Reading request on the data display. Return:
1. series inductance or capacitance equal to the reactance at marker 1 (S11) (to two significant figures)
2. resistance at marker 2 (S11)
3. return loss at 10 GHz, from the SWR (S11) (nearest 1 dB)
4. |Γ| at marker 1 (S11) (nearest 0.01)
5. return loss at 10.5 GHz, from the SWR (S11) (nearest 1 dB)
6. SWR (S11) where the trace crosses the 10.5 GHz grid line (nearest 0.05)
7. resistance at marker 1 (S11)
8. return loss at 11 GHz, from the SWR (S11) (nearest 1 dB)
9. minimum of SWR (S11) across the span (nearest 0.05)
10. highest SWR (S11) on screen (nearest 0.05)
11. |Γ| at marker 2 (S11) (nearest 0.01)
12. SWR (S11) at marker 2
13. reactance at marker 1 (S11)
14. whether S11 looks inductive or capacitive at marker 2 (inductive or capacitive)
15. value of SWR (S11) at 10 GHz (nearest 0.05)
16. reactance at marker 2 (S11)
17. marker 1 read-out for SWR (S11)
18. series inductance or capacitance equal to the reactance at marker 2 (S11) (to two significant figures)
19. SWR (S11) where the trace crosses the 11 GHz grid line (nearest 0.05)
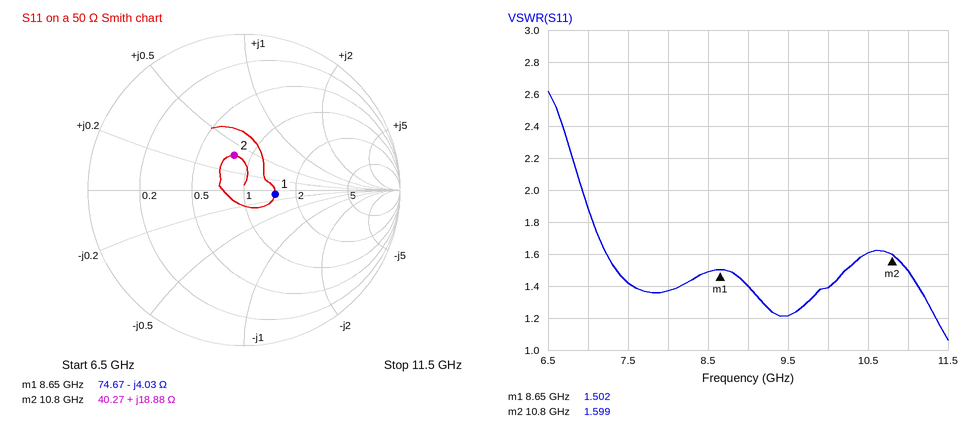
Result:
4.6 pF
40.27 Ω
16 dB
0.20
13 dB
1.60
74.67 Ω
14 dB
1.05
2.60
0.23
1.599
-4.03 Ω
inductive
1.40
+18.88 Ω
1.502
280 pH
1.50
